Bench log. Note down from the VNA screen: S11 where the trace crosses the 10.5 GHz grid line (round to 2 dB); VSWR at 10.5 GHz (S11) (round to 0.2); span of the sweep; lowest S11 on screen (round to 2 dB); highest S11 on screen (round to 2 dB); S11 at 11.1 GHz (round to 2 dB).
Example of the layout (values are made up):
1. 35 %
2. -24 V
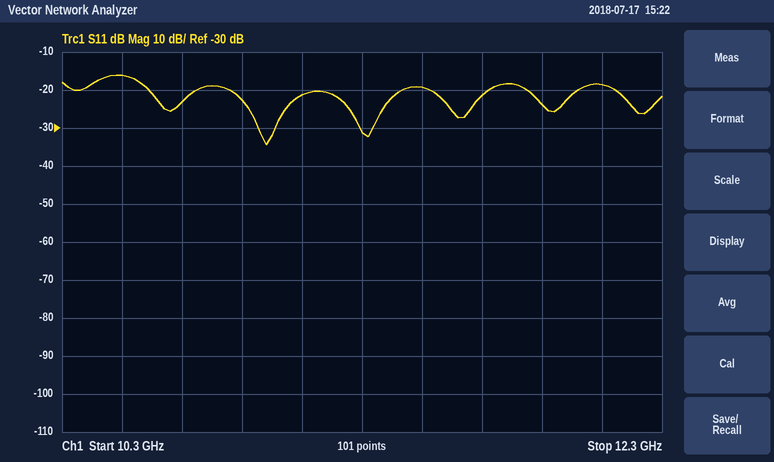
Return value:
1. -16 dB
2. 1.4
3. 2 GHz
4. -34 dB
5. -16 dB
6. -22 dB
